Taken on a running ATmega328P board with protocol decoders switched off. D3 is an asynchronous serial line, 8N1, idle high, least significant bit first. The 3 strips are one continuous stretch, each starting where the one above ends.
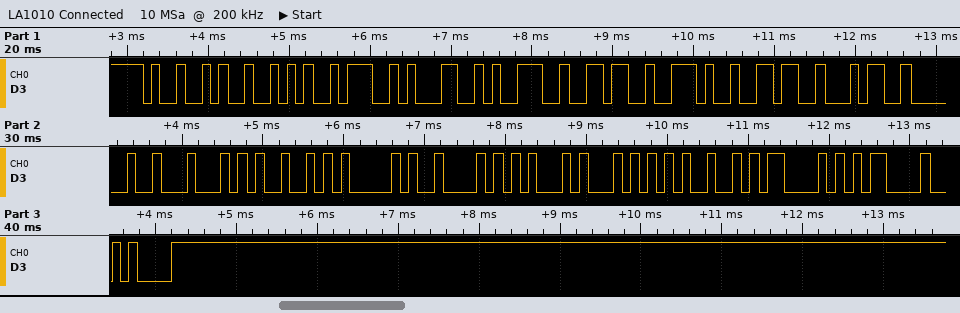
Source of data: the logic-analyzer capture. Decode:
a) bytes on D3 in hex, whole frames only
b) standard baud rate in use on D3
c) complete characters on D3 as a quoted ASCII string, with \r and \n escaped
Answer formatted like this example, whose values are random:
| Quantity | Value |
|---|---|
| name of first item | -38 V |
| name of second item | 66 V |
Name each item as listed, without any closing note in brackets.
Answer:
| Quantity | Value |
|---|---|
| bytes on D3 in hex, whole frames only | 0x49 0x52 0x3A 0x31 0x39 0x36 0x2E 0x36 0x34 0x20 0x44 0x49 0x41 0x42 0x45 0x54 0x49 0x43 0x0D 0x0A |
| standard baud rate in use on D3 | 9600 baud |
| complete characters on D3 as a quoted ASCII string, with \r and \n escaped | "IR:196.64 DIABETIC\r\n" |
